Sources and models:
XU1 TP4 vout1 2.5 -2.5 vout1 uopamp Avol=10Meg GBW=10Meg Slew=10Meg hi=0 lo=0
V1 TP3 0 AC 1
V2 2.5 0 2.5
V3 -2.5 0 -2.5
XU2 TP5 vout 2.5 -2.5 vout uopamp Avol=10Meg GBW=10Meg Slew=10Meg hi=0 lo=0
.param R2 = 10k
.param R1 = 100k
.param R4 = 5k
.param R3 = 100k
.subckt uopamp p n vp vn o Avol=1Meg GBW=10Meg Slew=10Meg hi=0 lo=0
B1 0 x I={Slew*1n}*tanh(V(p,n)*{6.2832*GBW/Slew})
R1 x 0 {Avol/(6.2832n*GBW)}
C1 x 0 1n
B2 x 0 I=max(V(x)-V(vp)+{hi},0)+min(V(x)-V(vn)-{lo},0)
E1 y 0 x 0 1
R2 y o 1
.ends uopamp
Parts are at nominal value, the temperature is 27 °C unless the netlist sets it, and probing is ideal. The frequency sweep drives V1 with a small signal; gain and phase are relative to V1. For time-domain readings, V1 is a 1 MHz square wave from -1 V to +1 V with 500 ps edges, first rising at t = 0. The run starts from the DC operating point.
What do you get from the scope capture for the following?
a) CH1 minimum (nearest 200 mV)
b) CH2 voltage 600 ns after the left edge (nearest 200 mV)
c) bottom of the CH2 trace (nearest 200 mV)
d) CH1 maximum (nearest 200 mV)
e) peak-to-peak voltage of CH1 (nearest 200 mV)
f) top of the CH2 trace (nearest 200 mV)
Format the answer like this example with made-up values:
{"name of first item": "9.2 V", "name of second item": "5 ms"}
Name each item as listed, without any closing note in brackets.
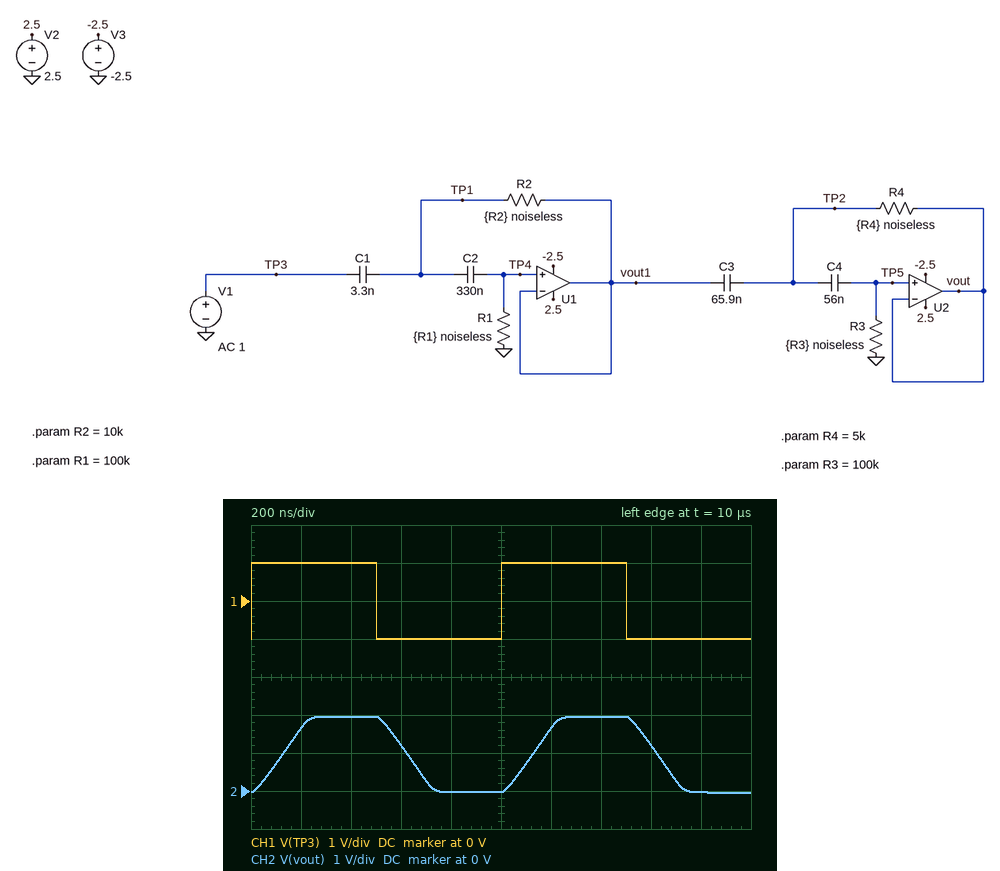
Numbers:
{"CH1 minimum": "-1.0 V", "CH2 voltage 600 ns after the left edge": "1.2 V", "bottom of the CH2 trace": "0 V", "CH1 maximum": "1.0 V", "peak-to-peak voltage of CH1": "2.0 V", "top of the CH2 trace": "2.0 V"}
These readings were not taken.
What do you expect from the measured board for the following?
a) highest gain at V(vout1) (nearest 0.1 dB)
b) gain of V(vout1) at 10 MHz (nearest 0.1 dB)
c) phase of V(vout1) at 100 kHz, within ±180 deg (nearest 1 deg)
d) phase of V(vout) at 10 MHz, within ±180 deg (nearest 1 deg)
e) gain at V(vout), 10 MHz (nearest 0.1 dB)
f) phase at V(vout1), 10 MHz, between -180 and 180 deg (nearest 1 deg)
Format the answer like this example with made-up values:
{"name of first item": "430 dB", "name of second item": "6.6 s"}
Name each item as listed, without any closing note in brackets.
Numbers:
{"highest gain at V(vout1)": "0 dB", "gain of V(vout1) at 10 MHz": "-3.0 dB", "phase of V(vout1) at 100 kHz, within ±180 deg": "0 deg", "phase of V(vout) at 10 MHz, within ±180 deg": "-90 deg", "gain at V(vout), 10 MHz": "-6.0 dB", "phase at V(vout1), 10 MHz, between -180 and 180 deg": "-45 deg"}
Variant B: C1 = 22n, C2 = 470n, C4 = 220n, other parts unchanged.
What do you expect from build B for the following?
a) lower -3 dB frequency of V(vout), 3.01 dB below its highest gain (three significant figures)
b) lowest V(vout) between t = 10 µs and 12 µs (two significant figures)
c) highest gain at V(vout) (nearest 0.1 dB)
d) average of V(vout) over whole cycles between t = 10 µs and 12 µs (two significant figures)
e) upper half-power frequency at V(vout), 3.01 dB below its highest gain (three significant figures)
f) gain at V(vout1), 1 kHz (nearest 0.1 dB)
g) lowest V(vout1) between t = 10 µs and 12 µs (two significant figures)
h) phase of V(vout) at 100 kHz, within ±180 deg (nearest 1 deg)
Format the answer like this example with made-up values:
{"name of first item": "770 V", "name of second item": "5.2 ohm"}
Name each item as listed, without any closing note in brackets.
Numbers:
{"lower -3 dB frequency of V(vout), 3.01 dB below its highest gain": "53.5 Hz", "lowest V(vout) between t = 10 µs and 12 µs": "-8.1 mV", "highest gain at V(vout)": "4.0 dB", "average of V(vout) over whole cycles between t = 10 µs and 12 µs": "990 mV", "upper half-power frequency at V(vout), 3.01 dB below its highest gain": "151 Hz", "gain at V(vout1), 1 kHz": "0 dB", "lowest V(vout1) between t = 10 µs and 12 µs": "-5.7 mV", "phase of V(vout) at 100 kHz, within ±180 deg": "-1 deg"}
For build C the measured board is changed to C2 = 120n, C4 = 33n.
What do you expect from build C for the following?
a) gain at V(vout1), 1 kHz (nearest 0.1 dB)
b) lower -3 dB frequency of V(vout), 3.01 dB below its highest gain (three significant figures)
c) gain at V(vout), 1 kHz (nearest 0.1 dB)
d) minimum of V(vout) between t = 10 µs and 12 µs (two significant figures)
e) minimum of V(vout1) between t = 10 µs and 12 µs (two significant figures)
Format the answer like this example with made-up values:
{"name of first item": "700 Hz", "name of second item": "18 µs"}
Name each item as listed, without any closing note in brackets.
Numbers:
{"gain at V(vout1), 1 kHz": "-0.5 dB", "lower -3 dB frequency of V(vout), 3.01 dB below its highest gain": "191 Hz", "gain at V(vout), 1 kHz": "-0.3 dB", "minimum of V(vout) between t = 10 µs and 12 µs": "-42 mV", "minimum of V(vout1) between t = 10 µs and 12 µs": "-37 mV"}
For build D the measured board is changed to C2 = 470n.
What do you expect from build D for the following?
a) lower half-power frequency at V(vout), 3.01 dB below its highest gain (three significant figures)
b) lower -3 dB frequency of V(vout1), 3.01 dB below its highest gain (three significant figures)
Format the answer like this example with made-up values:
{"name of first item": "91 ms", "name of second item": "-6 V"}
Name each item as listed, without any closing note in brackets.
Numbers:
{"lower half-power frequency at V(vout), 3.01 dB below its highest gain": "386 Hz", "lower -3 dB frequency of V(vout1), 3.01 dB below its highest gain": "452 Hz"}
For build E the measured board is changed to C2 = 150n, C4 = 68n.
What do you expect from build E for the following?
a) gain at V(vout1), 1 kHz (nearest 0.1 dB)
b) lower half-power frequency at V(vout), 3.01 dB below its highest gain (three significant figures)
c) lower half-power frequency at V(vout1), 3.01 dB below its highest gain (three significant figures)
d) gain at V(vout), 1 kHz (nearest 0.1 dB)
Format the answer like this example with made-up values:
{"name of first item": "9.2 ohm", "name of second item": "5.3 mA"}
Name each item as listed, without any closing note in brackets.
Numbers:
{"gain at V(vout1), 1 kHz": "-0.6 dB", "lower half-power frequency at V(vout), 3.01 dB below its highest gain": "342 Hz", "lower half-power frequency at V(vout1), 3.01 dB below its highest gain": "396 Hz", "gain at V(vout), 1 kHz": "-0.5 dB"}
